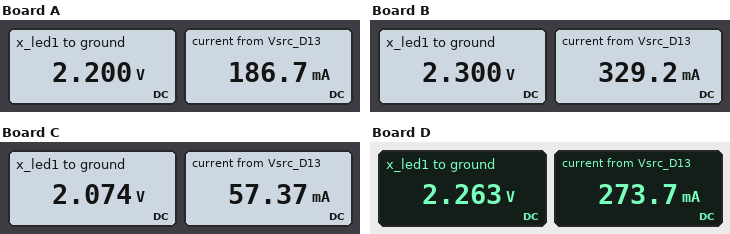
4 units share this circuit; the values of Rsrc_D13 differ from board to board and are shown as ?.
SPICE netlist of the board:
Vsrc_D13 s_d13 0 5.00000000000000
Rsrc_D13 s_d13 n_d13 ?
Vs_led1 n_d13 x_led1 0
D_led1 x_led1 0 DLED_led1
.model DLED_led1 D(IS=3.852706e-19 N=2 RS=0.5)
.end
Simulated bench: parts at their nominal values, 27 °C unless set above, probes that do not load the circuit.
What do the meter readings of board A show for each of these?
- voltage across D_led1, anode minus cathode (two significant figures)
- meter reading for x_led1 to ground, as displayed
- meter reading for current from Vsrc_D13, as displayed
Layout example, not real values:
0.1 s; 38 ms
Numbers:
2.2 V; 2.200 V; 186.7 mA
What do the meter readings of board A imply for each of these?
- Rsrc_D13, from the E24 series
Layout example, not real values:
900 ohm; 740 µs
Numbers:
15 Ω
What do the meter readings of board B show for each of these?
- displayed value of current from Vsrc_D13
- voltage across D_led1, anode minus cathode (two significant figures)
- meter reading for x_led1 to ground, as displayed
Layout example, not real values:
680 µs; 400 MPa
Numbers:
329.2 mA; 2.3 V; 2.300 V
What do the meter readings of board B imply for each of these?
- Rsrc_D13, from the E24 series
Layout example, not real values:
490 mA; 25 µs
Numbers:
8.2 Ω
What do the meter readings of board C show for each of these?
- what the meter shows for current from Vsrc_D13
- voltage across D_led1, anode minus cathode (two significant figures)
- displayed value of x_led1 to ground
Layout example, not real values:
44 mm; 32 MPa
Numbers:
57.37 mA; 2.1 V; 2.074 V
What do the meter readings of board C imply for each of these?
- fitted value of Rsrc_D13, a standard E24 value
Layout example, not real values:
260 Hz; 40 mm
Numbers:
51 Ω
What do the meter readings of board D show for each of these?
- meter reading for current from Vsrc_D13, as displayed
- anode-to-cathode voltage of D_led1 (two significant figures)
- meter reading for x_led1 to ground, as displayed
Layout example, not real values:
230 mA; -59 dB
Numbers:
273.7 mA; 2.3 V; 2.263 V
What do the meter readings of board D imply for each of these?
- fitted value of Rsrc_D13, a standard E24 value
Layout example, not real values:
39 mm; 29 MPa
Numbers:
10 Ω
